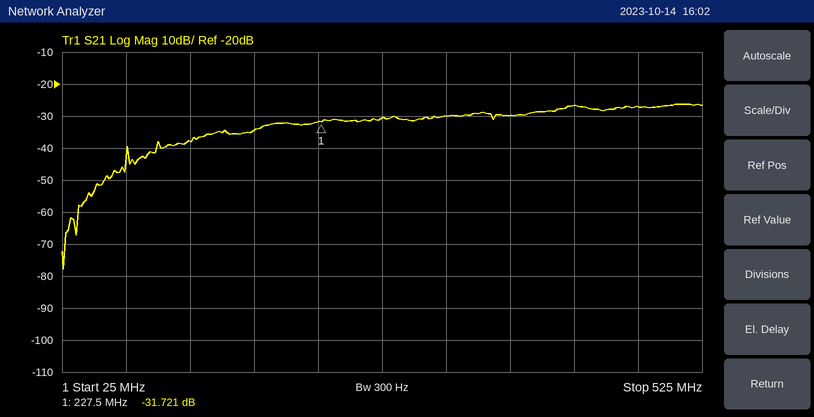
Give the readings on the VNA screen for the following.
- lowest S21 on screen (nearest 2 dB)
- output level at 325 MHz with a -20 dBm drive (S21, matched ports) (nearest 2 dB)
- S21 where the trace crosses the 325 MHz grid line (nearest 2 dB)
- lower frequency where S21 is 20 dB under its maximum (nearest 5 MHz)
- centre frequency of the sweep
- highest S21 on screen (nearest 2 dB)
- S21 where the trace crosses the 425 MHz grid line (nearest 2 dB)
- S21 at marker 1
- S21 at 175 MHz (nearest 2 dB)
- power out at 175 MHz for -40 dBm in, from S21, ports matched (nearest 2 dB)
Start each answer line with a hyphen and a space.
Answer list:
- -78 dB
- -50 dBm
- -30 dB
- 75 MHz
- 275 MHz
- -26 dB
- -26 dB
- -31.721 dB
- -34 dB
- -74 dBm
